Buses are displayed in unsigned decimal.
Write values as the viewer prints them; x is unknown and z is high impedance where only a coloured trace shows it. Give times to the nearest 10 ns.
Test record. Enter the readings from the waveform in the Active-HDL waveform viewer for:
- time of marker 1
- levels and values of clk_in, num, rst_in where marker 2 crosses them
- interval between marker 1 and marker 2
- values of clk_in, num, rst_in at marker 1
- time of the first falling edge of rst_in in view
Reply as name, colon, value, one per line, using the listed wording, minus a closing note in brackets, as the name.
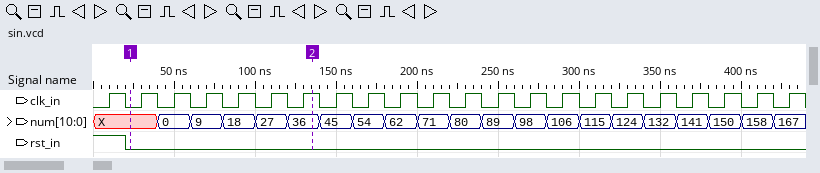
time of marker 1: 20 ns
levels and values of clk_in, num, rst_in where marker 2 crosses them: clk_in=1, num=36, rst_in=0
interval between marker 1 and marker 2: 110 ns
values of clk_in, num, rst_in at marker 1: clk_in=0, num=X, rst_in=0
time of the first falling edge of rst_in in view: 20 ns
